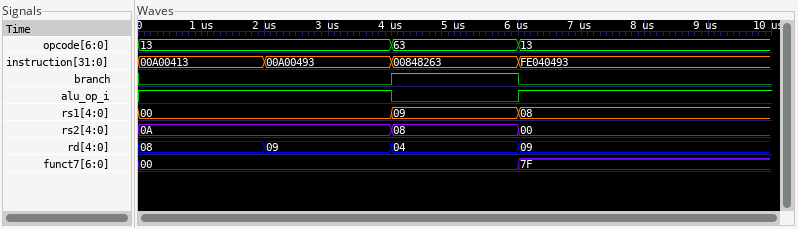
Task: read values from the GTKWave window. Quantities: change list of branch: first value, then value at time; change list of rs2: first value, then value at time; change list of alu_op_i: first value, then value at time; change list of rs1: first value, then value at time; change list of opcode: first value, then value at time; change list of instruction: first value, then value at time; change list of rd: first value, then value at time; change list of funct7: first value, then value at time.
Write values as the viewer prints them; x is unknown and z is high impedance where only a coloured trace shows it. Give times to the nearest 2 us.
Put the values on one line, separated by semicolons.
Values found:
0, 1 at 4 us, 0 at 6 us; 0A, 08 at 4 us, 00 at 6 us; 1, 0 at 4 us, 1 at 6 us; 00, 09 at 4 us, 08 at 6 us; 13, 63 at 4 us, 13 at 6 us; 00A00413, 00A00493 at 2 us, 00848263 at 4 us, FE040493 at 6 us; 08, 09 at 2 us, 04 at 4 us, 09 at 6 us; 00, 7F at 6 us
